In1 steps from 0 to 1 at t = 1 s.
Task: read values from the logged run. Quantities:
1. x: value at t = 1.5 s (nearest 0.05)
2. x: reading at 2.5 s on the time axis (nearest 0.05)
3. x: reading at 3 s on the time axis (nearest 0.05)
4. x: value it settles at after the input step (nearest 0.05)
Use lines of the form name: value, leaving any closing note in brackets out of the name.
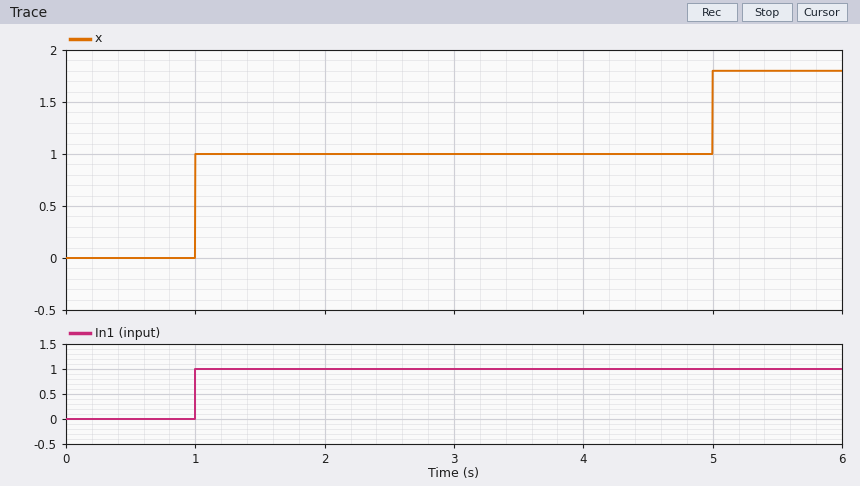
x: value at t = 1.5 s: 1.00
x: reading at 2.5 s on the time axis: 1.00
x: reading at 3 s on the time axis: 1.00
x: value it settles at after the input step: 1.80
